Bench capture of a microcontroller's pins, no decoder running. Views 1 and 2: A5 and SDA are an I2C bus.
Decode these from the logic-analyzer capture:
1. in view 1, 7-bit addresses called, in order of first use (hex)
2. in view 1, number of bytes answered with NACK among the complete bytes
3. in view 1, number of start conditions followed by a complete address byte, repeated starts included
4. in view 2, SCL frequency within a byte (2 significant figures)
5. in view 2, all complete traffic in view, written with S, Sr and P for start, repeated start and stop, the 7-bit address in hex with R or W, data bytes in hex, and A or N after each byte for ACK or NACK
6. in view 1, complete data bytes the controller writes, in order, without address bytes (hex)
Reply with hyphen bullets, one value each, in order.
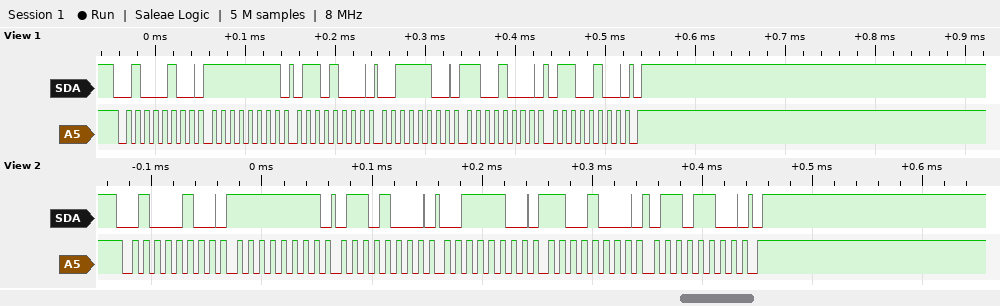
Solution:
- 0x22
- 0
- 1
- 100 kHz
- S 22W A FF A 68 A 3C A C8 A 6C A P
- FF 68 3C C8 64
